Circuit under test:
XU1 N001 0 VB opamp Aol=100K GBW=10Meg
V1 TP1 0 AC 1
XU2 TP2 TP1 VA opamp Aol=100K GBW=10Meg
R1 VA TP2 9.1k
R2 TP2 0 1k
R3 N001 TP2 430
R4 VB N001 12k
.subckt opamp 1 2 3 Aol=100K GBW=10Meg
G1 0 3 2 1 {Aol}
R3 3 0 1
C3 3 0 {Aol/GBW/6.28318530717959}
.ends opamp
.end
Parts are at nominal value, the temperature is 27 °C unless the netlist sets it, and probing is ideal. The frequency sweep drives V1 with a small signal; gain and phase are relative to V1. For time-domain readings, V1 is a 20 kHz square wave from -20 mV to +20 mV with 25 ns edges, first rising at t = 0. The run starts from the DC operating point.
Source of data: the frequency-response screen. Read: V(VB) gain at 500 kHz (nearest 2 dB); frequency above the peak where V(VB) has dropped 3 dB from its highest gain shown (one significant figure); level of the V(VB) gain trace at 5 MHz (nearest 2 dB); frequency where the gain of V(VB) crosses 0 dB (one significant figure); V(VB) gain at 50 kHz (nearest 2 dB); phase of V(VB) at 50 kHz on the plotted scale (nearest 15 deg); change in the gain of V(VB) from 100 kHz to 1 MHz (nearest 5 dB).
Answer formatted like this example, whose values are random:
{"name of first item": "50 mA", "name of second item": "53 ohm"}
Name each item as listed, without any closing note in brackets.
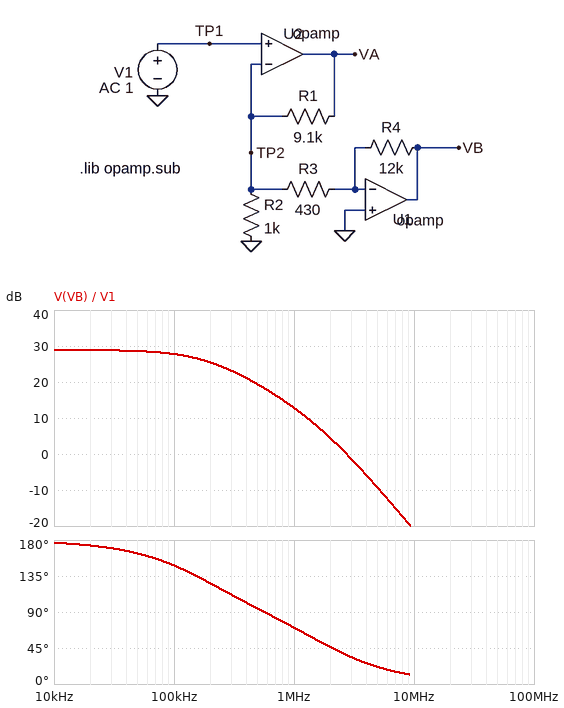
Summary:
{"V(VB) gain at 500 kHz": "20 dB", "frequency above the peak where V(VB) has dropped 3 dB from its highest gain shown": "200 kHz", "level of the V(VB) gain trace at 5 MHz": "-10 dB", "frequency where the gain of V(VB) crosses 0 dB": "3 MHz", "V(VB) gain at 50 kHz": "28 dB", "phase of V(VB) at 50 kHz on the plotted scale": "165 deg", "change in the gain of V(VB) from 100 kHz to 1 MHz": "-15 dB"}
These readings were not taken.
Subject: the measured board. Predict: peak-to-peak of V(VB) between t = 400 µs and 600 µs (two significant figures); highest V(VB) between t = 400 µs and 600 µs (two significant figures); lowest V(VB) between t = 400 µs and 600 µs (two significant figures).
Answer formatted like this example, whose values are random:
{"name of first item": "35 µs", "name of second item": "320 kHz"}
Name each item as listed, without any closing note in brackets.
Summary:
{"peak-to-peak of V(VB) between t = 400 µs and 600 µs": "1.1 V", "highest V(VB) between t = 400 µs and 600 µs": "560 mV", "lowest V(VB) between t = 400 µs and 600 µs": "-560 mV"}
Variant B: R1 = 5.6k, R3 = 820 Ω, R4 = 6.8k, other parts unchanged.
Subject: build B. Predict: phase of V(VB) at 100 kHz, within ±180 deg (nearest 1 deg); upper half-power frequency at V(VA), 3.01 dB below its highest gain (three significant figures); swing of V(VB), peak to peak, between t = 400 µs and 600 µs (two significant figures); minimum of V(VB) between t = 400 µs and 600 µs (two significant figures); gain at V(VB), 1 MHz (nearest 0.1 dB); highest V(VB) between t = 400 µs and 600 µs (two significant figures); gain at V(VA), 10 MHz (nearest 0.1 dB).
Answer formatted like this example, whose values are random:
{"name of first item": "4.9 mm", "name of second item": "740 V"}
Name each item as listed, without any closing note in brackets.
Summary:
{"phase of V(VB) at 100 kHz, within ±180 deg": "167 deg", "upper half-power frequency at V(VA), 3.01 dB below its highest gain": "541 kHz", "swing of V(VB), peak to peak, between t = 400 µs and 600 µs": "330 mV", "minimum of V(VB) between t = 400 µs and 600 µs": "-170 mV", "gain at V(VB), 1 MHz": "11.2 dB", "highest V(VB) between t = 400 µs and 600 µs": "170 mV", "gain at V(VA), 10 MHz": "-0.2 dB"}
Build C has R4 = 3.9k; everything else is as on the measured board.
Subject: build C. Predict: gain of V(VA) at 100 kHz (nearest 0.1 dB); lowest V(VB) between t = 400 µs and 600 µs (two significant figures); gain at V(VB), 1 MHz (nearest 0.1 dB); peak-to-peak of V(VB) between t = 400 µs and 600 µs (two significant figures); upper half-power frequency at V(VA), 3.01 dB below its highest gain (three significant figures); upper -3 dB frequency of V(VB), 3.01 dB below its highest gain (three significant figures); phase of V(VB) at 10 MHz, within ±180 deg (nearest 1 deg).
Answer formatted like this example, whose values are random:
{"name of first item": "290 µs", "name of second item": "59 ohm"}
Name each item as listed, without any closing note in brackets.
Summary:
{"gain of V(VA) at 100 kHz": "29.3 dB", "lowest V(VB) between t = 400 µs and 600 µs": "-180 mV", "gain at V(VB), 1 MHz": "6.8 dB", "peak-to-peak of V(VB) between t = 400 µs and 600 µs": "360 mV", "upper half-power frequency at V(VA), 3.01 dB below its highest gain": "263 kHz", "upper -3 dB frequency of V(VB), 3.01 dB below its highest gain": "261 kHz", "phase of V(VB) at 10 MHz, within ±180 deg": "19 deg"}
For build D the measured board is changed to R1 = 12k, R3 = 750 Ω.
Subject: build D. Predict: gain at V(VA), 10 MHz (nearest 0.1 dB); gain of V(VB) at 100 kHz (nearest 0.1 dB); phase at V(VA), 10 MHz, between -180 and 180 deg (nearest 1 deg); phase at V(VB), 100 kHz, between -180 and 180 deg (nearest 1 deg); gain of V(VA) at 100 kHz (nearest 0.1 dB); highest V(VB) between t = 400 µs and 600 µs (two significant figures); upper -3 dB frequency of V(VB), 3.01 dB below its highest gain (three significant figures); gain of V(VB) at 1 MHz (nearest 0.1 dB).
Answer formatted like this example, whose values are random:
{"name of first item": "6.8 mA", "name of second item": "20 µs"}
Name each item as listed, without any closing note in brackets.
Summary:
{"gain at V(VA), 10 MHz": "-0.1 dB", "gain of V(VB) at 100 kHz": "23.4 dB", "phase at V(VA), 10 MHz, between -180 and 180 deg": "-86 deg", "phase at V(VB), 100 kHz, between -180 and 180 deg": "155 deg", "gain of V(VA) at 100 kHz": "28.6 dB", "highest V(VB) between t = 400 µs and 600 µs": "320 mV", "upper -3 dB frequency of V(VB), 3.01 dB below its highest gain": "244 kHz", "gain of V(VB) at 1 MHz": "10.5 dB"}
